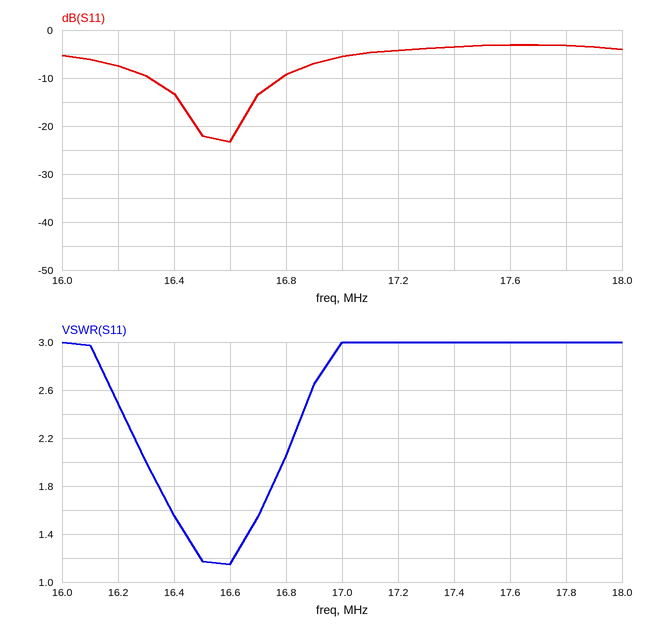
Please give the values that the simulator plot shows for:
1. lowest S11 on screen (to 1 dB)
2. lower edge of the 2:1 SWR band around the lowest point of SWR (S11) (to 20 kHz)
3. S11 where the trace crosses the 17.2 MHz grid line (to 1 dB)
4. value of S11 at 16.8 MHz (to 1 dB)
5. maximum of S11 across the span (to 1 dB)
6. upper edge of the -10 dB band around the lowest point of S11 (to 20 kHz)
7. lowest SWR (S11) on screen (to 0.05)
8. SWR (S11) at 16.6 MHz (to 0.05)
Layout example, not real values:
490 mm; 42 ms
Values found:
-23 dB; 16.30 MHz; -4 dB; -9 dB; -3 dB; 16.78 MHz; 1.15; 1.15
